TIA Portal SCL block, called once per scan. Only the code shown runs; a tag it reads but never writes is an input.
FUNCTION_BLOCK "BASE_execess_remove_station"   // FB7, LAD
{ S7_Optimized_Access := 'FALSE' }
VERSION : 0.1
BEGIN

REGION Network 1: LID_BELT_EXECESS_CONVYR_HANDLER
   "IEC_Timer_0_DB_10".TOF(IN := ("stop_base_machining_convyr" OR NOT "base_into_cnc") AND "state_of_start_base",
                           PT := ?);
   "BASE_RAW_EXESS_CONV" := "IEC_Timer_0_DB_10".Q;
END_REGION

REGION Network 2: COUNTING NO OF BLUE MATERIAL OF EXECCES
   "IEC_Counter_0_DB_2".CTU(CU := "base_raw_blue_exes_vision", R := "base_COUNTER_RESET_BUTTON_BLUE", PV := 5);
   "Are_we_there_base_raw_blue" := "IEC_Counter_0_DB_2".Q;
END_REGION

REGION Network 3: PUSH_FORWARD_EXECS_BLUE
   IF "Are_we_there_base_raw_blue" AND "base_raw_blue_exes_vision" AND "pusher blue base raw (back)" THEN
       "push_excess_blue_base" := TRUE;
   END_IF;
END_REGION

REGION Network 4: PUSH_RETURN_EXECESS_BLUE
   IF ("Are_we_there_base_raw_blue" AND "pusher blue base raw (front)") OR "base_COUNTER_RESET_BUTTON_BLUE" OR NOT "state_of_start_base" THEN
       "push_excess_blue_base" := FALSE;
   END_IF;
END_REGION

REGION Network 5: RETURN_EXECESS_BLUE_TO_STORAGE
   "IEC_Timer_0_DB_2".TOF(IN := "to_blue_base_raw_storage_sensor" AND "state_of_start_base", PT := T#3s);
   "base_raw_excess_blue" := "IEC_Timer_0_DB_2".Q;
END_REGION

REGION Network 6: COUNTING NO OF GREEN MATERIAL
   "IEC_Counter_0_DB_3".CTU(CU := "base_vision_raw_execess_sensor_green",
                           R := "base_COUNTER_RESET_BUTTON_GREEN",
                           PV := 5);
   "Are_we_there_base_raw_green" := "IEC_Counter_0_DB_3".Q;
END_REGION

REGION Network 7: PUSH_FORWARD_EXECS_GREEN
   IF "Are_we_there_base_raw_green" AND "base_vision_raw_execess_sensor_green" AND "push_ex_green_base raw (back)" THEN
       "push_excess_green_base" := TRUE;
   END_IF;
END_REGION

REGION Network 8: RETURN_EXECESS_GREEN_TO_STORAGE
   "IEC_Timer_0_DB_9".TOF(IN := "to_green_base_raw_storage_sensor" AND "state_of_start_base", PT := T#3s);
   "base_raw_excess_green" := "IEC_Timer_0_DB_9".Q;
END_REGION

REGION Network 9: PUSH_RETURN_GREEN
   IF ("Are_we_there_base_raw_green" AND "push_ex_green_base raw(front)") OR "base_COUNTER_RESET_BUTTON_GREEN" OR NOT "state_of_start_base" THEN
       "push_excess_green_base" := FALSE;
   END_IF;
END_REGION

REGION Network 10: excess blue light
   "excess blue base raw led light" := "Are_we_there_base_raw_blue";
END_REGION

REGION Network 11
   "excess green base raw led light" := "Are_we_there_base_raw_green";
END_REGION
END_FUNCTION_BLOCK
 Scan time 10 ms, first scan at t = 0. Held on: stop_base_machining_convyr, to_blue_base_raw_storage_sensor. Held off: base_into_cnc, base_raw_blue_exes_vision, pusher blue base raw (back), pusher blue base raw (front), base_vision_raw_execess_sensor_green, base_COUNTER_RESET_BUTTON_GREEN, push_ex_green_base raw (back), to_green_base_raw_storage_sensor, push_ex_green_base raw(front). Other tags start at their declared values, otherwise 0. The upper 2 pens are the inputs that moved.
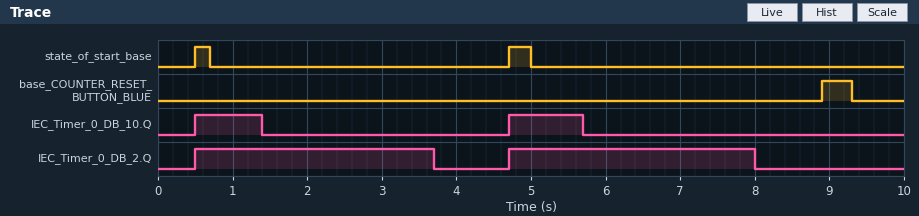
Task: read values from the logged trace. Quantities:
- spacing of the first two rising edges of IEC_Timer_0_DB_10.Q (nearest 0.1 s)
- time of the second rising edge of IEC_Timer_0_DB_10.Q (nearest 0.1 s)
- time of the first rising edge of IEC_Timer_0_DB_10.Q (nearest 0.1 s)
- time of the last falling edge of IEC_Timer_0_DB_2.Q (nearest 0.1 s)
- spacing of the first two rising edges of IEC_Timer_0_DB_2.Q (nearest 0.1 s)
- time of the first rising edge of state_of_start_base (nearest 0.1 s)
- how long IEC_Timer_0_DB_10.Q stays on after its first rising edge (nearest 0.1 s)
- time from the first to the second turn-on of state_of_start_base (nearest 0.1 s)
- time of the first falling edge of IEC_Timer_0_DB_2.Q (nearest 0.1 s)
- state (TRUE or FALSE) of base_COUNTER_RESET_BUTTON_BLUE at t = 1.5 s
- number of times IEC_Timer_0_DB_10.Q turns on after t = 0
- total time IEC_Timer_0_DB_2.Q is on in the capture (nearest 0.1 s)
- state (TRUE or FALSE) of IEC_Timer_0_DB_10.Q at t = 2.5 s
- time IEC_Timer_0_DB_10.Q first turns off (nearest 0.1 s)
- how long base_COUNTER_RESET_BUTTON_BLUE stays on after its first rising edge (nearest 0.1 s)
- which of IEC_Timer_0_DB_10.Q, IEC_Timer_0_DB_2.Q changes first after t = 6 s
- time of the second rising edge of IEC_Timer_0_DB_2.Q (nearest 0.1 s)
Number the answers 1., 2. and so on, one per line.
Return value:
1. 4.2 s
2. 4.7 s
3. 0.5 s
4. 8.0 s
5. 4.2 s
6. 0.5 s
7. 0.9 s
8. 4.2 s
9. 3.7 s
10. FALSE
11. 2
12. 6.5 s
13. FALSE
14. 1.4 s
15. 0.4 s
16. IEC_Timer_0_DB_2.Q
17. 4.7 s
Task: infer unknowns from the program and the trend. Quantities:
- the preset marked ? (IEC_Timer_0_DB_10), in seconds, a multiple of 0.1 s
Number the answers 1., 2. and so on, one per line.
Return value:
1. 0.7 s
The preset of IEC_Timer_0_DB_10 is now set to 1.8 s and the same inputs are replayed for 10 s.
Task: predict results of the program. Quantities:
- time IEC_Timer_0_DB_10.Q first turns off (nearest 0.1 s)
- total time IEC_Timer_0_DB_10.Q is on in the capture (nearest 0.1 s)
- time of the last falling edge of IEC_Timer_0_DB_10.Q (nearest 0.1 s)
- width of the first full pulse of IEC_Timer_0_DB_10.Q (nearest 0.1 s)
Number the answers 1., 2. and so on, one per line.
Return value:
1. 2.5 s
2. 4.1 s
3. 6.8 s
4. 2.0 s
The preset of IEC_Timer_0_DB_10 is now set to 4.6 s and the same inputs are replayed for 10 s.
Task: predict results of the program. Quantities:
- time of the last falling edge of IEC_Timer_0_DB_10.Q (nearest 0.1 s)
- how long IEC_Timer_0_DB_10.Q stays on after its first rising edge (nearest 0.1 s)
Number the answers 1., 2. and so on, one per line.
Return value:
1. 9.6 s
2. 9.1 s
